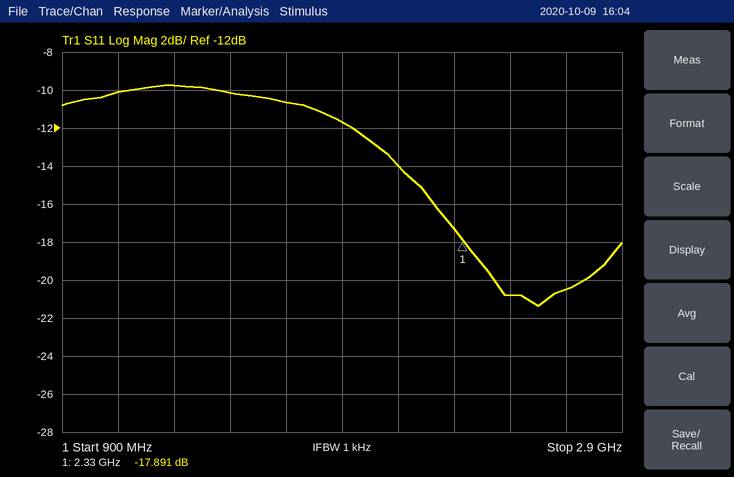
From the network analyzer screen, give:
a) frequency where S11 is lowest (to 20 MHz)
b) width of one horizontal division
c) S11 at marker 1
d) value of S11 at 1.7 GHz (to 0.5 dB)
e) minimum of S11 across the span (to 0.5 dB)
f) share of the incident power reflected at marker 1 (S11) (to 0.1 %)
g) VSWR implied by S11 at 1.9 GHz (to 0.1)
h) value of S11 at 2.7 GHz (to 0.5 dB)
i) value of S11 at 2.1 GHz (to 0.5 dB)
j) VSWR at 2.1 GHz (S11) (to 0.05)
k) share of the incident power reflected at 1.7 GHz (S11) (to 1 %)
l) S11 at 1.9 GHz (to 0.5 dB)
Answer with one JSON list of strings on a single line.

["2.60 GHz", "200 MHz", "-17.891 dB", "-10.5 dB", "-21.5 dB", "1.6 %", "1.7", "-20.5 dB", "-14.0 dB", "1.50", "9 %", "-11.5 dB"]
